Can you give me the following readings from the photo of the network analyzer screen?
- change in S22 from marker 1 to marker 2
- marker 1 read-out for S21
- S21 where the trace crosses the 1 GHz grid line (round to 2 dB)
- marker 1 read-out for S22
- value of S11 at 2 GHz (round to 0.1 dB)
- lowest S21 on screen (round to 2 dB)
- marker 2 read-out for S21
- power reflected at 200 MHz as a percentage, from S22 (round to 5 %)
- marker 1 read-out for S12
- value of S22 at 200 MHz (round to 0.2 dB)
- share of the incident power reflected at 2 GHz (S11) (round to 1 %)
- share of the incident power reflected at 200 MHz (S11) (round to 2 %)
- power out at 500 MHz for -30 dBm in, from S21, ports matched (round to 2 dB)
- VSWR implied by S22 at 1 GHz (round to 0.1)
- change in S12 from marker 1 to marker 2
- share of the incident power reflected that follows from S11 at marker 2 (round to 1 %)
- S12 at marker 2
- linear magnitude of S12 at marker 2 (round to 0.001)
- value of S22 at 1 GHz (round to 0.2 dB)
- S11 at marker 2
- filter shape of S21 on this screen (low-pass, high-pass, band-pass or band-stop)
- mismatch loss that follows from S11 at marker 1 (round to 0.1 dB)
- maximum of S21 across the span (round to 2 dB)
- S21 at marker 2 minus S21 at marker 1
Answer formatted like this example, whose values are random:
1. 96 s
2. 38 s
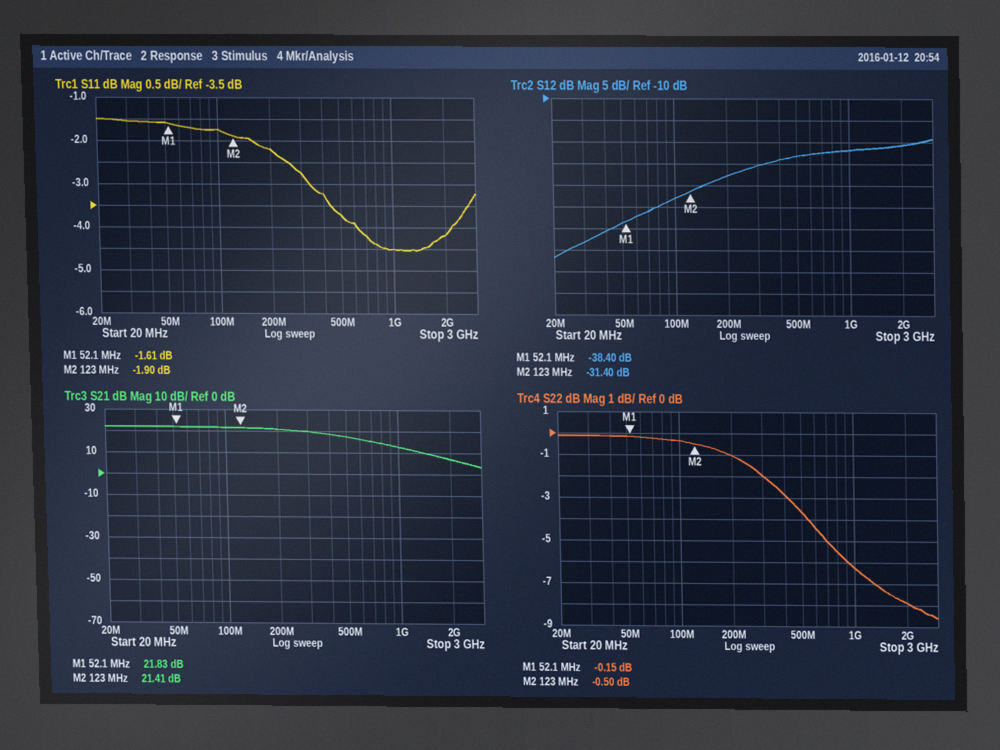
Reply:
1. -0.35 dB
2. 21.83 dB
3. 12 dB
4. -0.15 dB
5. -4.2 dB
6. 4 dB
7. 21.41 dB
8. 80 %
9. -38.40 dB
10. -1.0 dB
11. 38 %
12. 60 %
13. -12 dBm
14. 2.9
15. 7.00 dB
16. 65 %
17. -31.40 dB
18. 0.027
19. -6.2 dB
20. -1.90 dB
21. low-pass
22. 5.1 dB
23. 22 dB
24. -0.42 dB
